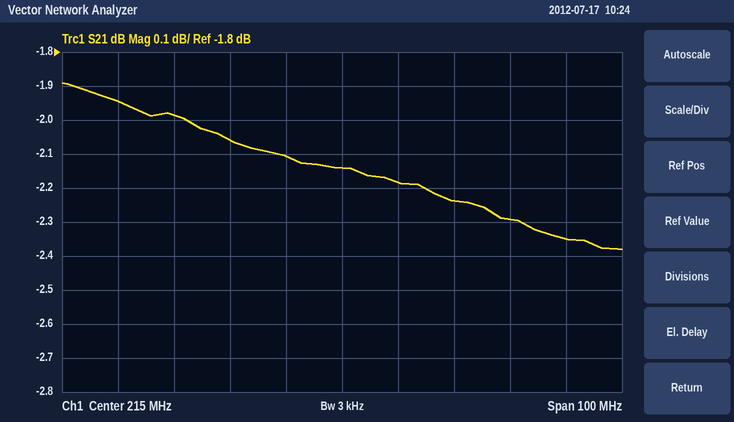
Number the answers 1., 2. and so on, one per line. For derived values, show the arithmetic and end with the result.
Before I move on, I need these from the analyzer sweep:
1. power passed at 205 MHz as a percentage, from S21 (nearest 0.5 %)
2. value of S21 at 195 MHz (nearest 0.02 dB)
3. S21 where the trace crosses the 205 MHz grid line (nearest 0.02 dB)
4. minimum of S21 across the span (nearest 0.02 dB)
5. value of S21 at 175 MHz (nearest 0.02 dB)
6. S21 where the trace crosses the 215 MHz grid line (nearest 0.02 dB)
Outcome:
1. 10^(-2.1/10) ≈ 61.7 %, so 61.5 % to the nearest 0.5 %
2. -2.06 dB
3. -2.10 dB
4. -2.38 dB
5. -1.94 dB
6. -2.14 dB
